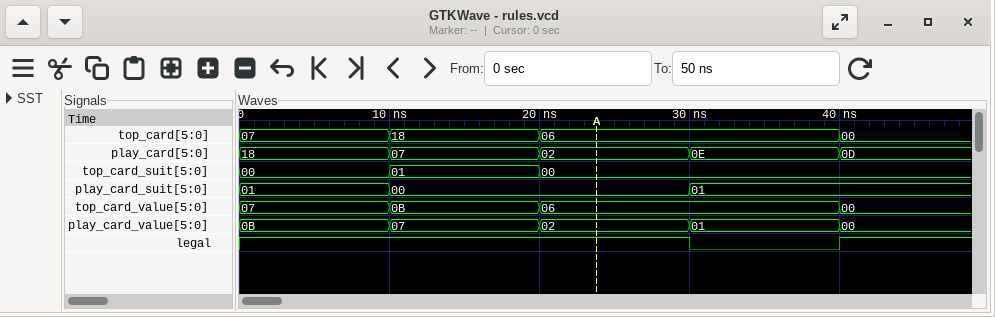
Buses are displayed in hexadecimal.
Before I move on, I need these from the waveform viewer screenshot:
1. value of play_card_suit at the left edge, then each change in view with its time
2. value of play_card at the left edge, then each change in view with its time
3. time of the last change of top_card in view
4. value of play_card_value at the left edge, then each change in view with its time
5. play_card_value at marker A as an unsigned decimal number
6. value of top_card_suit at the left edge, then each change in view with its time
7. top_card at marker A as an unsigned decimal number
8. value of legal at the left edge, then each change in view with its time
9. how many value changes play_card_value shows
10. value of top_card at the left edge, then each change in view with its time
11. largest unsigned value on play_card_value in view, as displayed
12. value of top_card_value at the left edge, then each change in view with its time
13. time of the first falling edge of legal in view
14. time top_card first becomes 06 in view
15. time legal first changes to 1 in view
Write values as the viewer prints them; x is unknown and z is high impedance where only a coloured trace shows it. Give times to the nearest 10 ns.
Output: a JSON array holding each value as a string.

["01, 00 at 10 ns, 01 at 30 ns", "18, 07 at 10 ns, 02 at 20 ns, 0E at 30 ns, 0D at 40 ns", "40 ns", "0B, 07 at 10 ns, 02 at 20 ns, 01 at 30 ns, 00 at 40 ns", "2", "00, 01 at 10 ns, 00 at 20 ns", "6", "1, 0 at 30 ns, 1 at 40 ns", "4", "07, 18 at 10 ns, 06 at 20 ns, 00 at 40 ns", "0B", "07, 0B at 10 ns, 06 at 20 ns, 00 at 40 ns", "30 ns", "20 ns", "40 ns"]
